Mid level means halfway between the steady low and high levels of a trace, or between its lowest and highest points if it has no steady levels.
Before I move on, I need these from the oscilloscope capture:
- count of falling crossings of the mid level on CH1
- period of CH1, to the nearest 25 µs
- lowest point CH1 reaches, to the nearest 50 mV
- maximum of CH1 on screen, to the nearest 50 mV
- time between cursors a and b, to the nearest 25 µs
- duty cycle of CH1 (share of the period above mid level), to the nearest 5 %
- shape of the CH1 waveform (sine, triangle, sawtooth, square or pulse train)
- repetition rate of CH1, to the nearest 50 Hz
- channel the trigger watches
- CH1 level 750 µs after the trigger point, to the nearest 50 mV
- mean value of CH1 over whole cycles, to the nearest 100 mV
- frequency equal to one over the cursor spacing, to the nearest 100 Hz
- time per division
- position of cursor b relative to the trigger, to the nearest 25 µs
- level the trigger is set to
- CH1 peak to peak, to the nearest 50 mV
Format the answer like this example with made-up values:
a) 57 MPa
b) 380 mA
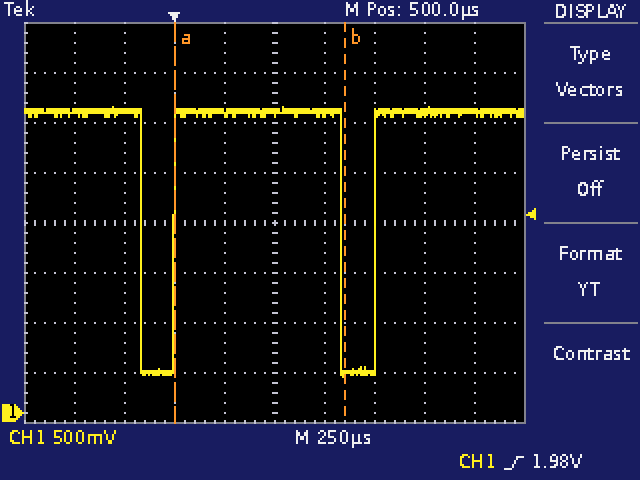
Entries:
a) 2
b) 1.000 ms
c) 350 mV
d) 3.05 V
e) 850 µs
f) 85 %
g) pulse train
h) 1.00 kHz
i) CH1
j) 3.00 V
k) 2.6 V
l) 1.2 kHz
m) 250 µs
n) +850 µs
o) 1.98 V
p) 2.70 V
